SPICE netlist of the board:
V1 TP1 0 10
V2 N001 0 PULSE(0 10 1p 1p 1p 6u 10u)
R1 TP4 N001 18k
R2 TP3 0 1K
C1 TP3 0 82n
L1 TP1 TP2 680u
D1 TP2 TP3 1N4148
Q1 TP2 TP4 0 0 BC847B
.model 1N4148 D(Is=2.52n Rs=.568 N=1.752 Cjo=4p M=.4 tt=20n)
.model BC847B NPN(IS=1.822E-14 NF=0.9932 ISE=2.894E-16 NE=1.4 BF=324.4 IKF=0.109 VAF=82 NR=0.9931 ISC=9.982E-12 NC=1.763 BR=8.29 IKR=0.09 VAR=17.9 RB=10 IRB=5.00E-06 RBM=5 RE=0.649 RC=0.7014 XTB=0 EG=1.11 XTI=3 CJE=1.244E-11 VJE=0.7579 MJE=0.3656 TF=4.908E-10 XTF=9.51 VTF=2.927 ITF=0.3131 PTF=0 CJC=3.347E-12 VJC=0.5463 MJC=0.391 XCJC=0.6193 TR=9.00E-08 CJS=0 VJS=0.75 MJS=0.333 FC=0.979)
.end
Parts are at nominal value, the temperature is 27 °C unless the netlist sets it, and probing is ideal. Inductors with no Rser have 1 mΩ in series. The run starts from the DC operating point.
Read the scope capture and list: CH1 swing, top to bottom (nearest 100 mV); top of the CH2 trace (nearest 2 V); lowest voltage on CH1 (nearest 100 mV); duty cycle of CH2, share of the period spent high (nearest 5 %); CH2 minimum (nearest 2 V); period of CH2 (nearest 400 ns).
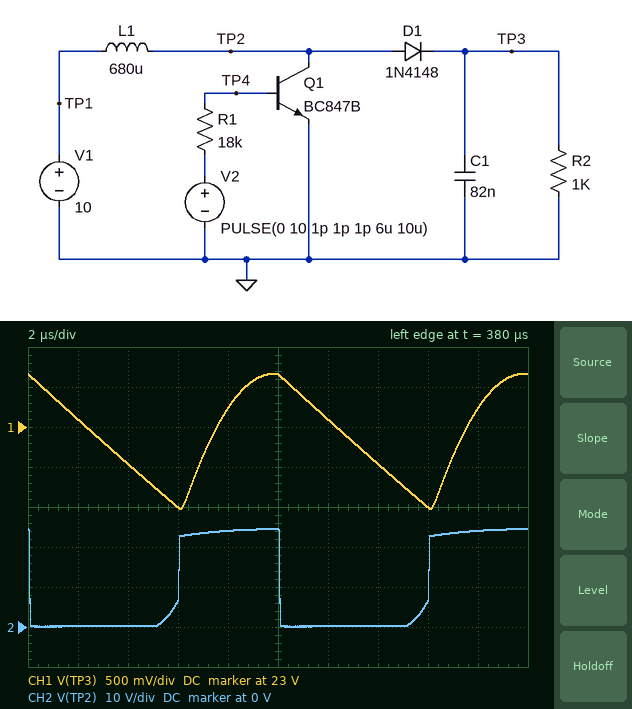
1.7 V
24 V
22.0 V
40 %
0 V
10.0 µs
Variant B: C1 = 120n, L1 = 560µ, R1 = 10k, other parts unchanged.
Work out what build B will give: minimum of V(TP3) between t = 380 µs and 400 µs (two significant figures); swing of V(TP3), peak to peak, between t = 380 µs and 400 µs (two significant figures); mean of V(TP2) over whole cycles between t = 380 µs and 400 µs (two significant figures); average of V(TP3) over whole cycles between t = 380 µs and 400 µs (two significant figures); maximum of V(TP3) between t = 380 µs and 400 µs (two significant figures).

24 V
1.3 V
10 V
25 V
26 V
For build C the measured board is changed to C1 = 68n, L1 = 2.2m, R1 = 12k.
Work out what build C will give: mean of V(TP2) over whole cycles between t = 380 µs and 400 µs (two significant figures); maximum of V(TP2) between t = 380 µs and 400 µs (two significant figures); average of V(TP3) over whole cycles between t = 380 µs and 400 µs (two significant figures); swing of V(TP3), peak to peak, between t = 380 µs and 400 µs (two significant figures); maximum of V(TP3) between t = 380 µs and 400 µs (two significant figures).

10 V
28 V
26 V
2.4 V
27 V
